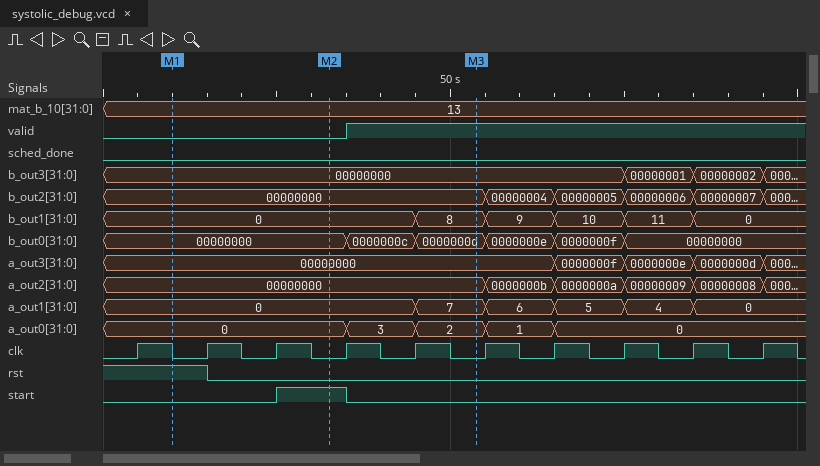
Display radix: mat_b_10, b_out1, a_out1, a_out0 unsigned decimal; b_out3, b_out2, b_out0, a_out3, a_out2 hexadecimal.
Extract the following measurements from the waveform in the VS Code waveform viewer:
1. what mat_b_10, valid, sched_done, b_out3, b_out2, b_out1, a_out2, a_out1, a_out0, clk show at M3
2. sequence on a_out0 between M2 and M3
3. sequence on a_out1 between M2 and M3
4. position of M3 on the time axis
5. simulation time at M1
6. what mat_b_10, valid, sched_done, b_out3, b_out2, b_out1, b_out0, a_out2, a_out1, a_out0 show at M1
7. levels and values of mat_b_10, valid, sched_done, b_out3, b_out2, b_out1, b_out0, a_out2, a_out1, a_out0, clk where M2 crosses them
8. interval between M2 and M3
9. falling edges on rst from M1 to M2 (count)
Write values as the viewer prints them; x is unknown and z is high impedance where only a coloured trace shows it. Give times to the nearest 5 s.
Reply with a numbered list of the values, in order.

1. mat_b_10=13, valid=1, sched_done=0, b_out3=00000000, b_out2=00000000, b_out1=8, a_out2=00000000, a_out1=7, a_out0=2, clk=0
2. 0, 3, 2
3. 0, 7
4. 55 s
5. 10 s
6. mat_b_10=13, valid=0, sched_done=0, b_out3=00000000, b_out2=00000000, b_out1=0, b_out0=00000000, a_out2=00000000, a_out1=0, a_out0=0
7. mat_b_10=13, valid=0, sched_done=0, b_out3=00000000, b_out2=00000000, b_out1=0, b_out0=00000000, a_out2=00000000, a_out1=0, a_out0=0, clk=0
8. 20 s
9. 1
